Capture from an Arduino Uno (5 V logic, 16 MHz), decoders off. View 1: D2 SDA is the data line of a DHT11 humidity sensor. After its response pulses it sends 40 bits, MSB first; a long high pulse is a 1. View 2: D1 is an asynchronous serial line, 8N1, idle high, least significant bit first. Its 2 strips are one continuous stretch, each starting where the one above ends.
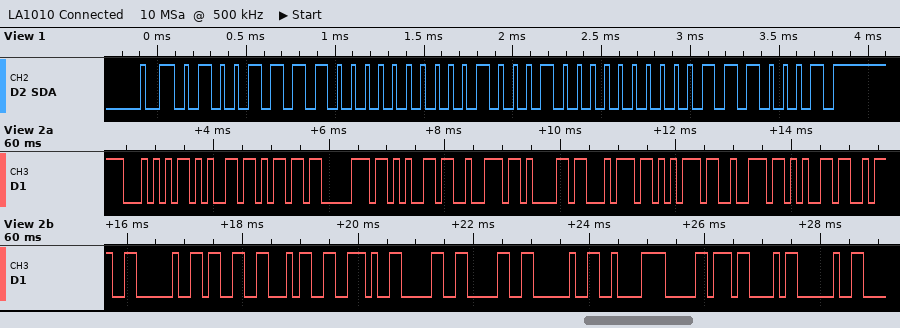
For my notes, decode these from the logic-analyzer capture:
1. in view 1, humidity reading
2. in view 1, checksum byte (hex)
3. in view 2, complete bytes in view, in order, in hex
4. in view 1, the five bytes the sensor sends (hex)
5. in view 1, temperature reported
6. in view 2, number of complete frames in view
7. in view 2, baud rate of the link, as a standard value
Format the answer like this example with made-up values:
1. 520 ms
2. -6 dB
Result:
1. 79 %
2. 0x71
3. 54 65 6D 70 65 72 61 74 75 72 65 3A 20 33 34 2E 30 30 20 C2 B0 43 20
4. 4F 00 22 00 71
5. 34.0 °C
6. 23
7. 9600 baud
